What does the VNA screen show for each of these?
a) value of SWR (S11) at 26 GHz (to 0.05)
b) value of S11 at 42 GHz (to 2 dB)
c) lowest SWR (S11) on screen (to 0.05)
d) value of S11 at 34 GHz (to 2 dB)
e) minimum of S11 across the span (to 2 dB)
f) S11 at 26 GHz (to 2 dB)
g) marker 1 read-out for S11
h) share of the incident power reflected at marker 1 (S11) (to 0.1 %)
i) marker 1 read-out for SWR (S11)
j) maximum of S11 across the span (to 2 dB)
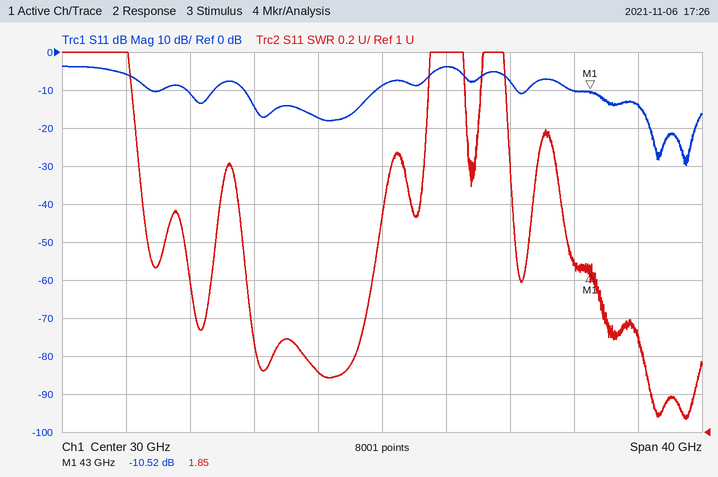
1.30
-10 dB
1.05
-4 dB
-30 dB
-18 dB
-10.52 dB
8.9 %
1.85
-4 dB
